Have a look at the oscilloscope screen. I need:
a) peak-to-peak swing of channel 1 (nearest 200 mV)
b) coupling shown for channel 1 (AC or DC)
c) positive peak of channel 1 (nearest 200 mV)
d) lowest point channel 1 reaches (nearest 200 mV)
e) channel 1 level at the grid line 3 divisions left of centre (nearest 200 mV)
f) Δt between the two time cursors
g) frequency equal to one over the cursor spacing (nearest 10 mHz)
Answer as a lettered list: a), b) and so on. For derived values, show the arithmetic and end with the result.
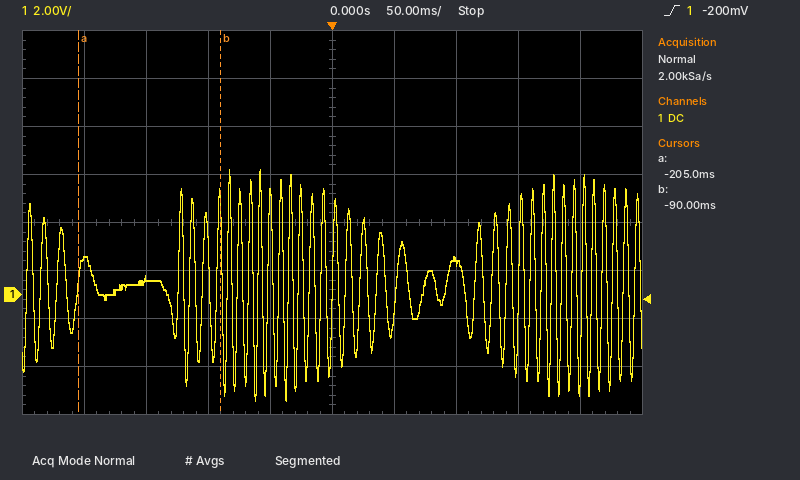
a) 5.2 V − (-4.4 V) = 9.6 V
b) DC
c) 5.2 V
d) -4.4 V
e) 600 mV
f) -90 ms − (-205 ms) = 115 ms
g) 1 / 115 ms ≈ 8.70 Hz
